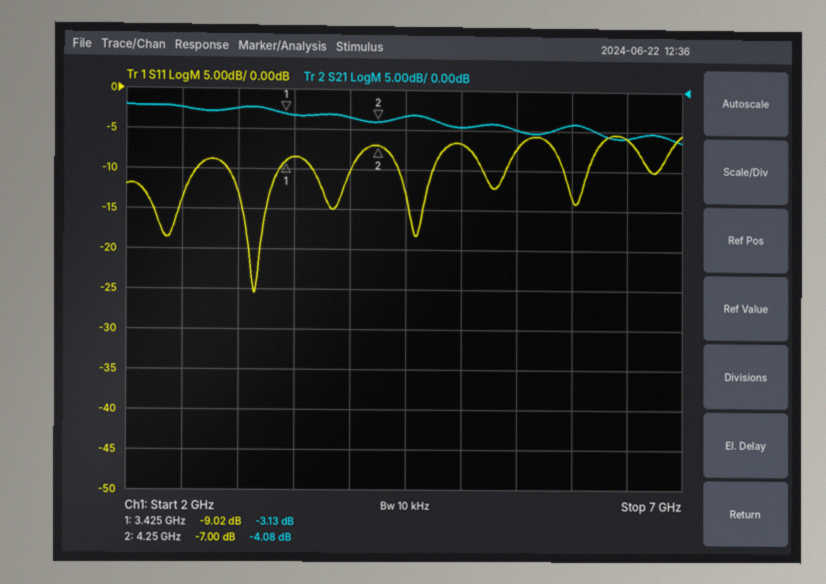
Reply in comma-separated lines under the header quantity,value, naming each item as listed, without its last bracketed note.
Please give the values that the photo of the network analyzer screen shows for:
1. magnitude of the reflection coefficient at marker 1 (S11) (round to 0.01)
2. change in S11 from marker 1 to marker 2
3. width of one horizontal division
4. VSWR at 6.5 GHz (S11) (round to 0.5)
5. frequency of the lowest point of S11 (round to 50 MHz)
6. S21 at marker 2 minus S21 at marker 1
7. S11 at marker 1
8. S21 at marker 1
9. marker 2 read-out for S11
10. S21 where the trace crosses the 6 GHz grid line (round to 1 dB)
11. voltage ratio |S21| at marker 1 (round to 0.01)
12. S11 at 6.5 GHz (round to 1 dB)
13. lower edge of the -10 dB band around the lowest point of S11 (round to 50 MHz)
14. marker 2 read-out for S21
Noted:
quantity,value
magnitude of the reflection coefficient at marker 1 (S11),0.35
change in S11 from marker 1 to marker 2,2.02 dB
width of one horizontal division,500 MHz
VSWR at 6.5 GHz (S11),3.0
frequency of the lowest point of S11,3.15 GHz
S21 at marker 2 minus S21 at marker 1,-0.95 dB
S11 at marker 1,-9.02 dB
S21 at marker 1,-3.13 dB
marker 2 read-out for S11,-7.00 dB
S21 where the trace crosses the 6 GHz grid line,-4 dB
voltage ratio |S21| at marker 1,0.70
S11 at 6.5 GHz,-6 dB
lower edge of the -10 dB band around the lowest point of S11,2.90 GHz
marker 2 read-out for S21,-4.08 dB
